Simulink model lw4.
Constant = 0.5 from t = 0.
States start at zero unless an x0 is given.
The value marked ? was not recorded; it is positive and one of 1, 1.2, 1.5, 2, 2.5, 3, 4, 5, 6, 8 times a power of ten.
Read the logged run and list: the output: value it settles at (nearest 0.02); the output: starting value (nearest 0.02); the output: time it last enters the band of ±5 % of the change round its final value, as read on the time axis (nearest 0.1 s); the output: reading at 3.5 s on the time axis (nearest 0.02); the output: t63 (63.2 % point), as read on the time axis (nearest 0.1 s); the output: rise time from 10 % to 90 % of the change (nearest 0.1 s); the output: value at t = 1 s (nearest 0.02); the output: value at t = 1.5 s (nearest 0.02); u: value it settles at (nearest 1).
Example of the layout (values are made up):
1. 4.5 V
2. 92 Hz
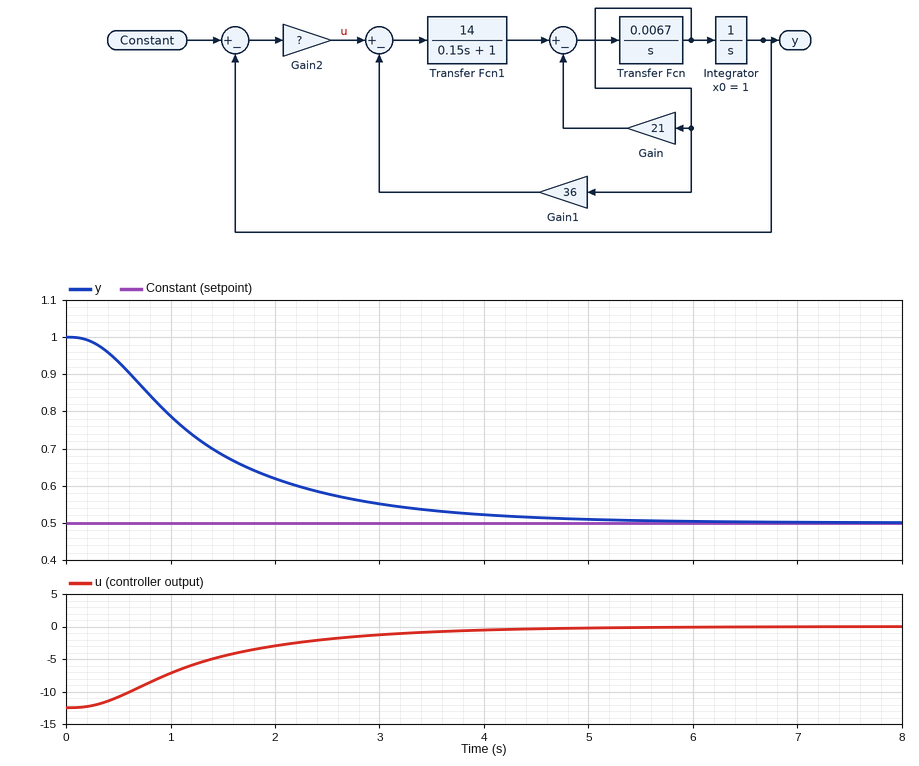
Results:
1. 0.50
2. 1.00
3. 3.8 s
4. 0.54
5. 1.5 s
6. 2.6 s
7. 0.78
8. 0.68
9. 0
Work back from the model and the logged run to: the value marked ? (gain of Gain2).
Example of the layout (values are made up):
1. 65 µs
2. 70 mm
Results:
1. 25
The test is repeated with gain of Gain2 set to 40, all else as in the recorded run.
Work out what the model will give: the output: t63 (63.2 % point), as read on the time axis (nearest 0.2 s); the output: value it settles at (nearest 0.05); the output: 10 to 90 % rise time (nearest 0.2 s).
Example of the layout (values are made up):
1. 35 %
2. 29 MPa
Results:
1. 1.0 s
2. 0.50
3. 1.2 s
